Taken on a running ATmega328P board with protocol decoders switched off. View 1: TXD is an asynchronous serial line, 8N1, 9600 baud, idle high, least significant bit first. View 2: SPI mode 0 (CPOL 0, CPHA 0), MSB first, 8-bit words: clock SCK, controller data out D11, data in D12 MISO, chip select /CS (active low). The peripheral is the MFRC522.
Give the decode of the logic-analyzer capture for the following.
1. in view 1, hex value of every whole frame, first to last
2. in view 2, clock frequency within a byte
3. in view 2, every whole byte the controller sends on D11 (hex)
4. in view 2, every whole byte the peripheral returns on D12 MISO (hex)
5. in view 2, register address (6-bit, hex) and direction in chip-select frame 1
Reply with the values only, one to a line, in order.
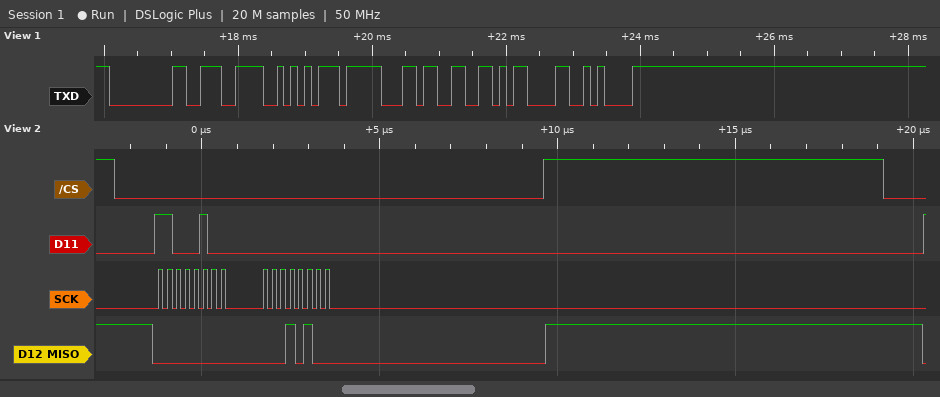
00 CE AA 1F 33 0D 0A
4 MHz
C4 00
00 14
0x22 read
